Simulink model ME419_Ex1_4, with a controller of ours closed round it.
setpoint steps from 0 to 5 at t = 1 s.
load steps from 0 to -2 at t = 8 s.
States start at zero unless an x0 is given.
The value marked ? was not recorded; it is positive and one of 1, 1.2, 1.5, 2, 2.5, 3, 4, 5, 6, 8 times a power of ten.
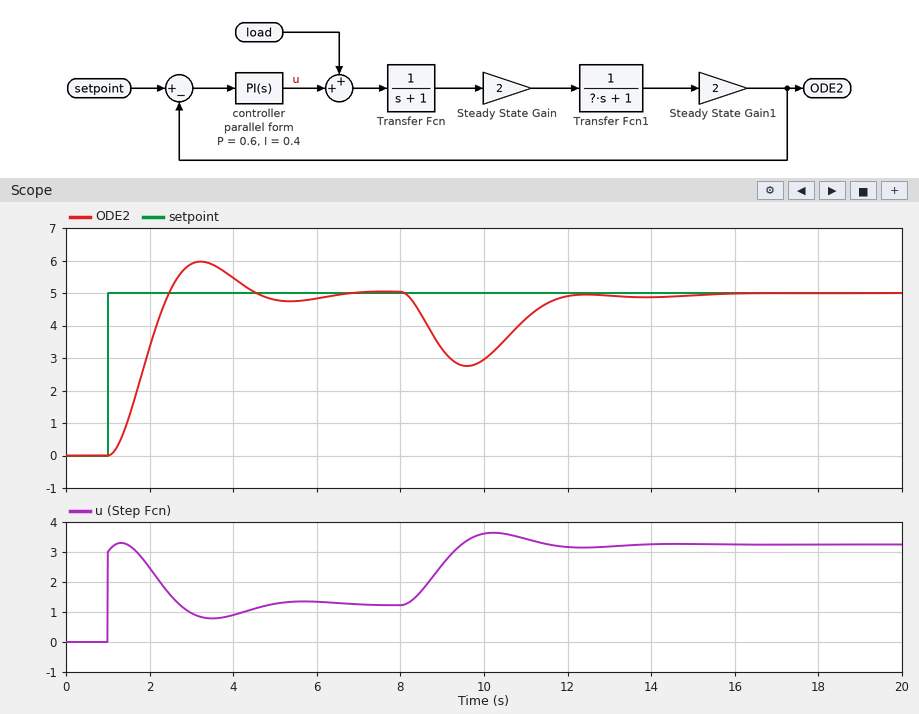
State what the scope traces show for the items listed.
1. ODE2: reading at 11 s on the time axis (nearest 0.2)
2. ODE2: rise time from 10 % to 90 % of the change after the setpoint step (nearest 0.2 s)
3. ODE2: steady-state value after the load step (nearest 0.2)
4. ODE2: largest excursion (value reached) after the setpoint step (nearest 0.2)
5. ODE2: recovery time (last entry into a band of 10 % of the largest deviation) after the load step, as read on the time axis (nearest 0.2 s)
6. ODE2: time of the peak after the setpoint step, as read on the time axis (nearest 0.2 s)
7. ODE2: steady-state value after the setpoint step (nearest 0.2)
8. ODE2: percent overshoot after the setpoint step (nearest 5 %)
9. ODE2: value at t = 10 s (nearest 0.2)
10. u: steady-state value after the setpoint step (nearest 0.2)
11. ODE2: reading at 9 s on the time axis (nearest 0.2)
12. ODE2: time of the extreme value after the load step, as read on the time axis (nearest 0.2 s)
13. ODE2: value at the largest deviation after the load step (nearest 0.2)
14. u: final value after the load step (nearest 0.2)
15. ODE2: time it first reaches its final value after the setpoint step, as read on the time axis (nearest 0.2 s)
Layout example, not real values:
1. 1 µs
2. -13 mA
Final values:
1. 4.2
2. 1.0 s
3. 5.0
4. 6.0
5. 11.6 s
6. 3.2 s
7. 5.0
8. 20 %
9. 3.0
10. 1.2
11. 3.2
12. 9.6 s
13. 2.8
14. 3.2
15. 2.4 s
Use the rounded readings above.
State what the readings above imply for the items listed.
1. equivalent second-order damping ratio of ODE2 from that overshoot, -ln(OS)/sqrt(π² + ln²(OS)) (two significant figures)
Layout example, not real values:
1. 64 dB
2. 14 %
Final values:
1. 0.46
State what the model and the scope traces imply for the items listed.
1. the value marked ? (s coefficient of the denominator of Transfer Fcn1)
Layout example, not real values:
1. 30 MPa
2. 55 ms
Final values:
1. 1
